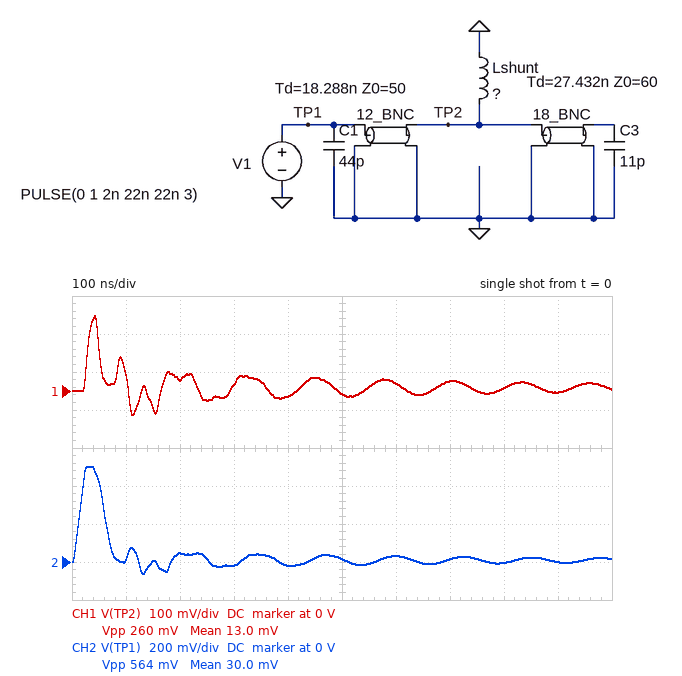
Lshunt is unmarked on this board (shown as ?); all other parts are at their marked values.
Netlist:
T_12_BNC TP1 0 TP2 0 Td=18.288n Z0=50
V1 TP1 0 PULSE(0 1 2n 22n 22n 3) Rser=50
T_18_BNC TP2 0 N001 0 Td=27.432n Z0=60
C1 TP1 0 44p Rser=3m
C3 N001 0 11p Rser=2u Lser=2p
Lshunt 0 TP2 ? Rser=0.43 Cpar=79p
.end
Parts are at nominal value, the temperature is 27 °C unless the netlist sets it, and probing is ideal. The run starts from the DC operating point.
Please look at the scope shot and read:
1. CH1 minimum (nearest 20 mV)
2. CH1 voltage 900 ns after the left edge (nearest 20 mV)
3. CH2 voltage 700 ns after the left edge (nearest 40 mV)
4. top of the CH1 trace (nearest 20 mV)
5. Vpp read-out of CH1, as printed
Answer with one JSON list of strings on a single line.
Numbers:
["-60 mV", "0 V", "0 V", "200 mV", "260 mV"]
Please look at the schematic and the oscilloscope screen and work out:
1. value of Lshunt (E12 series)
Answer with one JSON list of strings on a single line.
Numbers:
["220 nH"]
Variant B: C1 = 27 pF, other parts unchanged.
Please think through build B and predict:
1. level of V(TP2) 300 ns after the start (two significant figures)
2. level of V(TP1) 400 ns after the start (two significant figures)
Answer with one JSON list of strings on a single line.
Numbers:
["19 mV", "-19 mV"]
